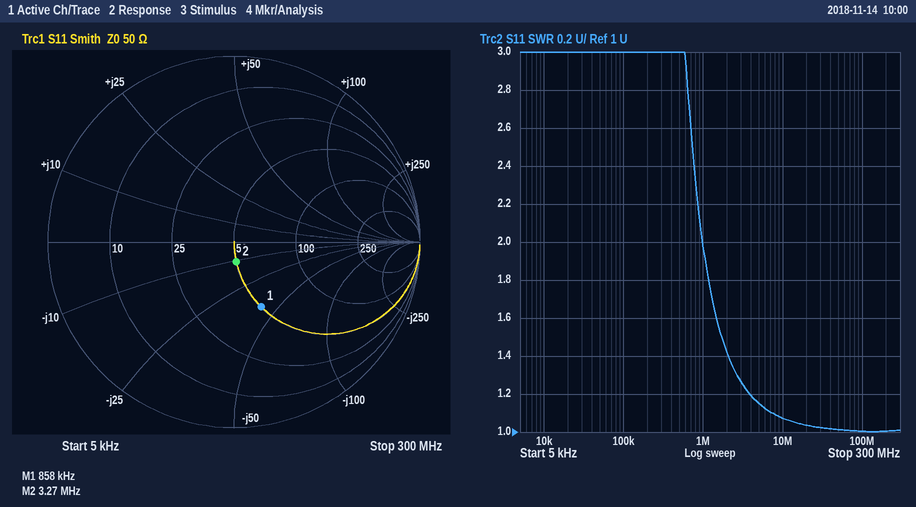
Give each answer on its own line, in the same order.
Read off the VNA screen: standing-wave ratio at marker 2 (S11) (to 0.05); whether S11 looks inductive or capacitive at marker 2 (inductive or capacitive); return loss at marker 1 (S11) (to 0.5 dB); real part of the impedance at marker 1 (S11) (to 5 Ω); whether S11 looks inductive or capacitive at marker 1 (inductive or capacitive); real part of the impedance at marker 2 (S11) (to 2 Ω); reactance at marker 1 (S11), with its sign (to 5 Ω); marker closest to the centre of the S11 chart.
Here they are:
1.25
capacitive
8.5 dB
50 Ω
capacitive
50 Ω
-40 Ω
marker 2
